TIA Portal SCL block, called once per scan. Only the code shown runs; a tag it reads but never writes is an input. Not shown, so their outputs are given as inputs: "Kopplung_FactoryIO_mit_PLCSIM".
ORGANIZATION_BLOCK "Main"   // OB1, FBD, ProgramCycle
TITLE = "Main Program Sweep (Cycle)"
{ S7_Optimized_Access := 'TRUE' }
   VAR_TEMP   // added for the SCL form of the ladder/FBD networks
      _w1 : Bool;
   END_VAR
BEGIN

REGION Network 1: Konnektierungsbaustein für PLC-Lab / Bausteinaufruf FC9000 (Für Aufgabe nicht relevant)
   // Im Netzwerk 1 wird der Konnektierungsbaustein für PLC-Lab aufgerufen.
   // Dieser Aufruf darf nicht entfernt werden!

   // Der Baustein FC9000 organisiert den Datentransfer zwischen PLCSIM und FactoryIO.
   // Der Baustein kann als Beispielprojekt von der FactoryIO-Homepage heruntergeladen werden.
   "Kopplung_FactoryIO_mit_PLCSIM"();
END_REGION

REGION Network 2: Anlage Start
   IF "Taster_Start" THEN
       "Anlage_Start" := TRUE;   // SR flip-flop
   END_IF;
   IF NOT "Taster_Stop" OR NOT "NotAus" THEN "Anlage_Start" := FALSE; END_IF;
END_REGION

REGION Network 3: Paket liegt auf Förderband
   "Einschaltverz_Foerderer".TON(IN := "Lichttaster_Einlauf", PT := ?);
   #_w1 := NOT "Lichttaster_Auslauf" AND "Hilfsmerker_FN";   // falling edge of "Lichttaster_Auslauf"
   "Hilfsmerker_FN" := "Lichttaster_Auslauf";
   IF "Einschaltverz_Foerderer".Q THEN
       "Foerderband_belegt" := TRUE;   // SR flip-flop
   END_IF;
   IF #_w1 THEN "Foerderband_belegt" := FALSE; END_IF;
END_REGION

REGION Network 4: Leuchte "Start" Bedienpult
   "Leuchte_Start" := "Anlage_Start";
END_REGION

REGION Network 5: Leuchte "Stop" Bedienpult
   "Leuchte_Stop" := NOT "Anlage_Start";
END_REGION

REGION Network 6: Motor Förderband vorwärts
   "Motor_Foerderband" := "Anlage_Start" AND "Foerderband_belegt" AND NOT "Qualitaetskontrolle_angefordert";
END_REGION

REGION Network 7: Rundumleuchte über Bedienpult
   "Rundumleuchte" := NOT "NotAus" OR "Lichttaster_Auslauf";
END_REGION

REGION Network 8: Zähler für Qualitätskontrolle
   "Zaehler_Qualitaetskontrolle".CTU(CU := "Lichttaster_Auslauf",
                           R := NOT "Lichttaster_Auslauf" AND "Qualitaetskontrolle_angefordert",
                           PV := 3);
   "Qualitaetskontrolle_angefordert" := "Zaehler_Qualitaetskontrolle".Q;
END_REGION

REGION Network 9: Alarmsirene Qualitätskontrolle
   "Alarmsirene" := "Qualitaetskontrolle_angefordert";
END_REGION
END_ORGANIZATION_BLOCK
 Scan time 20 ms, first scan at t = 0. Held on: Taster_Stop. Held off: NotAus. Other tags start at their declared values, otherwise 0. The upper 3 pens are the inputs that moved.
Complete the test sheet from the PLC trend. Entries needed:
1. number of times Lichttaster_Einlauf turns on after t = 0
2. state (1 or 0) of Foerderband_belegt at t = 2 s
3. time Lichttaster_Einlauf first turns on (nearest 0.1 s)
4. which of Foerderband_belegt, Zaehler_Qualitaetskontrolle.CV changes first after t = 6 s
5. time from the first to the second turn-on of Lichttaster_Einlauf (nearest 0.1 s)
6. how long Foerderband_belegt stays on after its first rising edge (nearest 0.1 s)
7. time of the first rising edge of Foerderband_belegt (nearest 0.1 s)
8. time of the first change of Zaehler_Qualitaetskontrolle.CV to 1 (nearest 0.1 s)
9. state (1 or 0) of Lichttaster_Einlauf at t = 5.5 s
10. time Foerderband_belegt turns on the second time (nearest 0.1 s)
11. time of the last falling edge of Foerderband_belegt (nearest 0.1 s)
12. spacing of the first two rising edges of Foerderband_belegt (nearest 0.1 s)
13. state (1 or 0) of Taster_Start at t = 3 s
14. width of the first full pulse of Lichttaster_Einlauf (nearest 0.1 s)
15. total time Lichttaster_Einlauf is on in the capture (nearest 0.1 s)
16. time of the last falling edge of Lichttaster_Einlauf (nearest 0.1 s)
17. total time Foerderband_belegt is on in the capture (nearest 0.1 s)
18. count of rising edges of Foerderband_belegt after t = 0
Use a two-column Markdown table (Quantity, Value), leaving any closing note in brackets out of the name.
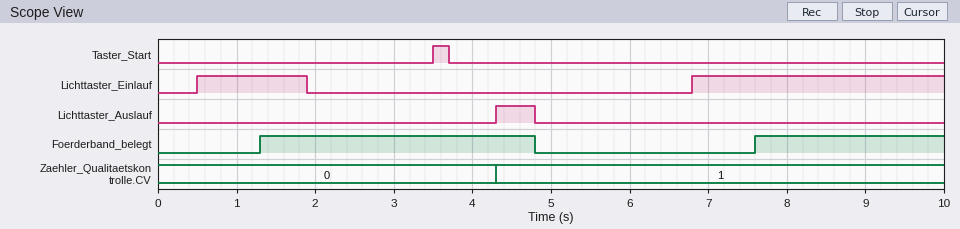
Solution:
| Quantity | Value |
|---|---|
| number of times Lichttaster_Einlauf turns on after t = 0 | 2 |
| state (1 or 0) of Foerderband_belegt at t = 2 s | 1 |
| time Lichttaster_Einlauf first turns on | 0.5 s |
| which of Foerderband_belegt, Zaehler_Qualitaetskontrolle.CV changes first after t = 6 s | Foerderband_belegt |
| time from the first to the second turn-on of Lichttaster_Einlauf | 6.3 s |
| how long Foerderband_belegt stays on after its first rising edge | 3.5 s |
| time of the first rising edge of Foerderband_belegt | 1.3 s |
| time of the first change of Zaehler_Qualitaetskontrolle.CV to 1 | 4.3 s |
| state (1 or 0) of Lichttaster_Einlauf at t = 5.5 s | 0 |
| time Foerderband_belegt turns on the second time | 7.6 s |
| time of the last falling edge of Foerderband_belegt | 4.8 s |
| spacing of the first two rising edges of Foerderband_belegt | 6.3 s |
| state (1 or 0) of Taster_Start at t = 3 s | 0 |
| width of the first full pulse of Lichttaster_Einlauf | 1.4 s |
| total time Lichttaster_Einlauf is on in the capture | 4.6 s |
| time of the last falling edge of Lichttaster_Einlauf | 1.9 s |
| total time Foerderband_belegt is on in the capture | 5.9 s |
| count of rising edges of Foerderband_belegt after t = 0 | 2 |
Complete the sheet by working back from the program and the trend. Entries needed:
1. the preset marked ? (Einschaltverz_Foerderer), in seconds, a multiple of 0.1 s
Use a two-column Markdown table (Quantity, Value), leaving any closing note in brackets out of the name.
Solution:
| Quantity | Value |
|---|---|
| the preset marked ? (Einschaltverz_Foerderer), in seconds, a multiple of 0.1 s | 0.8 s |
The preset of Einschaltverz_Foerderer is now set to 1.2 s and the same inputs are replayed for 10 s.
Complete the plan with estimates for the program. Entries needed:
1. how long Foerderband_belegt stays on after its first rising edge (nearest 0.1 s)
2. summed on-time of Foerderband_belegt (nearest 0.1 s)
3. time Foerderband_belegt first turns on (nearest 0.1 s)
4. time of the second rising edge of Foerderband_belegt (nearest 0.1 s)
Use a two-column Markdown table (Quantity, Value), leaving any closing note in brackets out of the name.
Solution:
| Quantity | Value |
|---|---|
| how long Foerderband_belegt stays on after its first rising edge | 3.1 s |
| summed on-time of Foerderband_belegt | 5.1 s |
| time Foerderband_belegt first turns on | 1.7 s |
| time of the second rising edge of Foerderband_belegt | 8.0 s |
